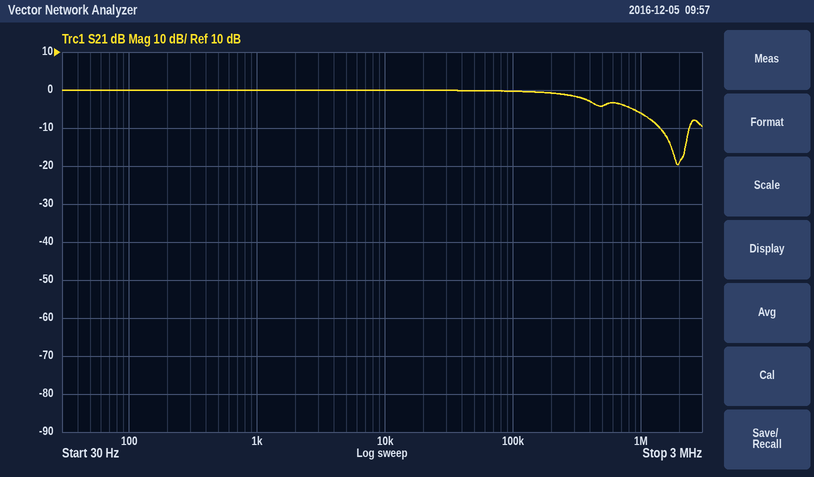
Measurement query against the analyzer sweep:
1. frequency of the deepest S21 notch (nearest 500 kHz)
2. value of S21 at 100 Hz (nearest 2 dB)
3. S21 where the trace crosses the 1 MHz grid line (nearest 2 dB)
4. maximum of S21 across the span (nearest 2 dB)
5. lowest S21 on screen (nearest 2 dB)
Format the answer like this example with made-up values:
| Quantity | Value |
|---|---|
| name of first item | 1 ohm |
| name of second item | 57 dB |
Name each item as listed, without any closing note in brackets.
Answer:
| Quantity | Value |
|---|---|
| frequency of the deepest S21 notch | 2.0 MHz |
| value of S21 at 100 Hz | 0 dB |
| S21 where the trace crosses the 1 MHz grid line | -6 dB |
| maximum of S21 across the span | 0 dB |
| lowest S21 on screen | -20 dB |
